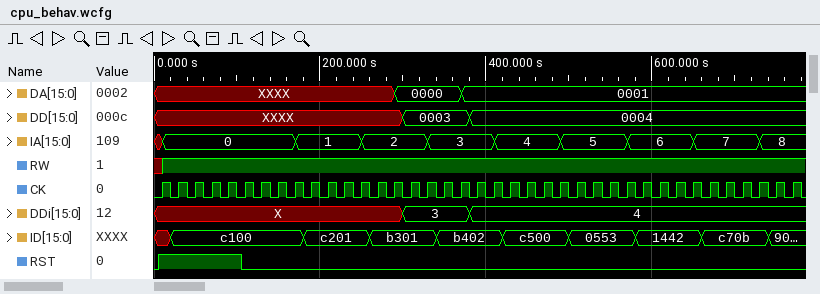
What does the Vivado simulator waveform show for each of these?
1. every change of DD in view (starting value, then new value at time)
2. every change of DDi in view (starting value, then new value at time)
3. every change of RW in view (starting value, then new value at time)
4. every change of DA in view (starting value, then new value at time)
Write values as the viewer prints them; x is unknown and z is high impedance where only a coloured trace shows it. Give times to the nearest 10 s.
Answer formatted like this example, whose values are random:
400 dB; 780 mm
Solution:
XXXX, 0003 at 300 s, 0004 at 380 s; X, 3 at 300 s, 4 at 380 s; x, 1 at 10 s; XXXX, 0000 at 290 s, 0001 at 370 s
